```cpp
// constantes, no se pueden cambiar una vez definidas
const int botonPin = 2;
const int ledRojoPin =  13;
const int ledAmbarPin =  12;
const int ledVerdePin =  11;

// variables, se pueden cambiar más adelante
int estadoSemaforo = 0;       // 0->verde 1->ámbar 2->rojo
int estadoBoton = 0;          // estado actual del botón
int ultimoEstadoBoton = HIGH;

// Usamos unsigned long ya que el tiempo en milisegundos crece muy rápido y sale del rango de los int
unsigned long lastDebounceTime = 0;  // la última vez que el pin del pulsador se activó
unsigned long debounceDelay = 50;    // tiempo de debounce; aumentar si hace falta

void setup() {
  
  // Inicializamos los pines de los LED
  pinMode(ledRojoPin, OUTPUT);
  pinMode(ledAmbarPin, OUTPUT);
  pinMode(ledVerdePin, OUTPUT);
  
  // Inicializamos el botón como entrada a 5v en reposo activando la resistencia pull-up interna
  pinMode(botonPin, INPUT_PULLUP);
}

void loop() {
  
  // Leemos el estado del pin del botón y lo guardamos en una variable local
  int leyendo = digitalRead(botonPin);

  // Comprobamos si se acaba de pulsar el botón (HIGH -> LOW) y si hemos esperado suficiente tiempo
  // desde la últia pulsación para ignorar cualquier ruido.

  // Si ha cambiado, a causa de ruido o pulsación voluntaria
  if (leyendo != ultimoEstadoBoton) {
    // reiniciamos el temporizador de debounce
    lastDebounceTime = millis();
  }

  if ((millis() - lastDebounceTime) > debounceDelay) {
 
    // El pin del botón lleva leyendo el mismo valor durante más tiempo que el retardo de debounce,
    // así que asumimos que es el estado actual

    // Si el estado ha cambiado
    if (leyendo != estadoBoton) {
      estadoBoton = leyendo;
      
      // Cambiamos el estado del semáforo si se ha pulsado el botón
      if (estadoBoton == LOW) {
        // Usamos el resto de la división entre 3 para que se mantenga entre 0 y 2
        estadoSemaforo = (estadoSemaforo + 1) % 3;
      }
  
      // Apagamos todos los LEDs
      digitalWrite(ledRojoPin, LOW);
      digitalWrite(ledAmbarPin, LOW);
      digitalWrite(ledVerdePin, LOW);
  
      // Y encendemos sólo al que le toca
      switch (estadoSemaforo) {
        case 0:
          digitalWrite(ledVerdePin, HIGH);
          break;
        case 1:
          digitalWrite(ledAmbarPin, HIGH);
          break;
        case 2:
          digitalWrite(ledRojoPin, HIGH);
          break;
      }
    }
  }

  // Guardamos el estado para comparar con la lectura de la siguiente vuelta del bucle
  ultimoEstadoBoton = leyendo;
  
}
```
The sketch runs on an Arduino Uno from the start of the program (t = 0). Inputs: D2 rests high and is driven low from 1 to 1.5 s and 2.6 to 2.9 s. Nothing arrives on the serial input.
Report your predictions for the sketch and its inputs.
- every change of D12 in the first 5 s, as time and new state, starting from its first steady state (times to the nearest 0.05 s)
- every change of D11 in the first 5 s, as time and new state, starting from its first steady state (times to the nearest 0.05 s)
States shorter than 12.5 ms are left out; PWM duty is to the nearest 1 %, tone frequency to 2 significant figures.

0 s low; 1.05 s high; 2.65 s low
0 s low; 0.05 s high; 1.05 s low
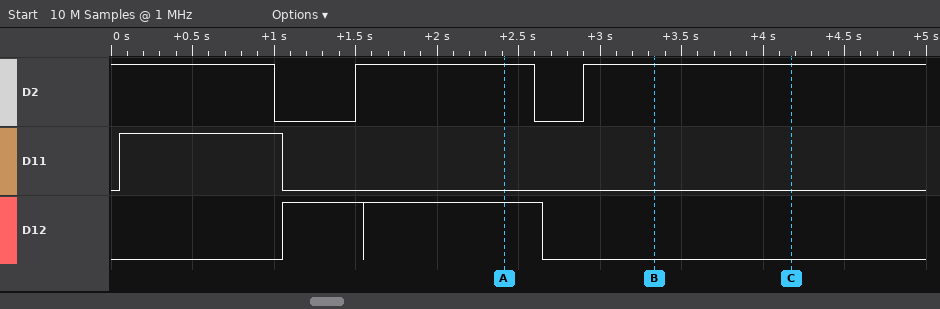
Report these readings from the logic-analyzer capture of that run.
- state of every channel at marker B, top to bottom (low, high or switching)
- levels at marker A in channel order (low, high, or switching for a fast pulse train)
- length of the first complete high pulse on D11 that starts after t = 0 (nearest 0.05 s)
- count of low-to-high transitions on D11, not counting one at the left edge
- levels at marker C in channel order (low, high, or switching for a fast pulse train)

D2 high, D11 low, D12 low
D2 high, D11 low, D12 high
1.00 s
1
D2 high, D11 low, D12 low
